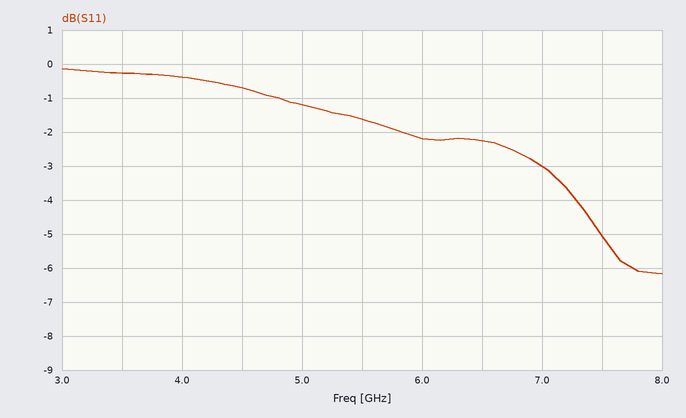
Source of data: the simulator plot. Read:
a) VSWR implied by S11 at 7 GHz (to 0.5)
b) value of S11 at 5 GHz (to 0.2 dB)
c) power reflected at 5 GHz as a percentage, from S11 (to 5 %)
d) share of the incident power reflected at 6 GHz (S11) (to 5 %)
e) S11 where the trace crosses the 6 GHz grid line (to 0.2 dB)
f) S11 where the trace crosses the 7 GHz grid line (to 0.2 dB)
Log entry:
6.0
-1.2 dB
75 %
60 %
-2.2 dB
-3.0 dB
